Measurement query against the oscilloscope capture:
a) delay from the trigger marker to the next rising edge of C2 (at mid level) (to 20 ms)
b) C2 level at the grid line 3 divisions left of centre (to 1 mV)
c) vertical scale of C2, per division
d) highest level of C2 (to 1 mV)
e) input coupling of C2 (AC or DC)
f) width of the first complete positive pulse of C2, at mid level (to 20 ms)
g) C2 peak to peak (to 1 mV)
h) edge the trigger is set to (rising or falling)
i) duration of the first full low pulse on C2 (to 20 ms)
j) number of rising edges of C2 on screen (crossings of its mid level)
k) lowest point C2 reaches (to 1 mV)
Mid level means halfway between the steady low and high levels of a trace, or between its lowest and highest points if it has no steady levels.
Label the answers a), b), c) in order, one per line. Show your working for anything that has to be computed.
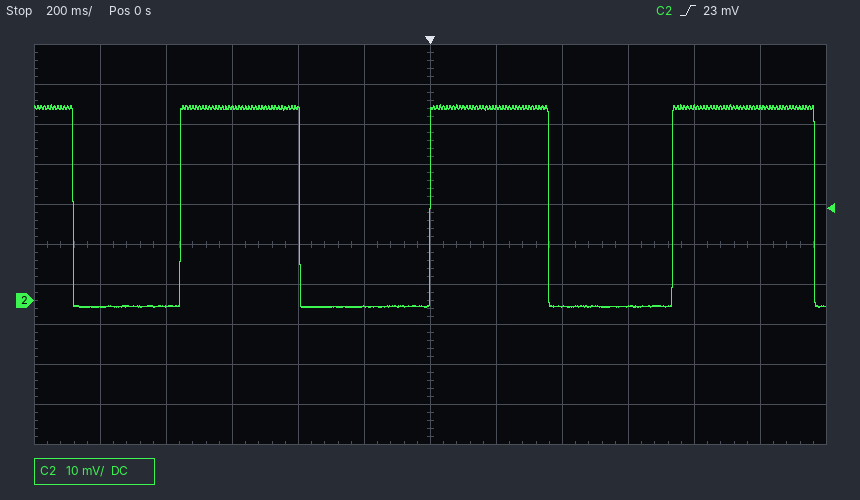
a) 740 ms
b) 48 mV
c) 10 mV
d) 49 mV
e) DC
f) 360 ms
g) 49 mV − (-2 mV) = 51 mV
h) rising
i) 320 ms
j) 3
k) -2 mV
